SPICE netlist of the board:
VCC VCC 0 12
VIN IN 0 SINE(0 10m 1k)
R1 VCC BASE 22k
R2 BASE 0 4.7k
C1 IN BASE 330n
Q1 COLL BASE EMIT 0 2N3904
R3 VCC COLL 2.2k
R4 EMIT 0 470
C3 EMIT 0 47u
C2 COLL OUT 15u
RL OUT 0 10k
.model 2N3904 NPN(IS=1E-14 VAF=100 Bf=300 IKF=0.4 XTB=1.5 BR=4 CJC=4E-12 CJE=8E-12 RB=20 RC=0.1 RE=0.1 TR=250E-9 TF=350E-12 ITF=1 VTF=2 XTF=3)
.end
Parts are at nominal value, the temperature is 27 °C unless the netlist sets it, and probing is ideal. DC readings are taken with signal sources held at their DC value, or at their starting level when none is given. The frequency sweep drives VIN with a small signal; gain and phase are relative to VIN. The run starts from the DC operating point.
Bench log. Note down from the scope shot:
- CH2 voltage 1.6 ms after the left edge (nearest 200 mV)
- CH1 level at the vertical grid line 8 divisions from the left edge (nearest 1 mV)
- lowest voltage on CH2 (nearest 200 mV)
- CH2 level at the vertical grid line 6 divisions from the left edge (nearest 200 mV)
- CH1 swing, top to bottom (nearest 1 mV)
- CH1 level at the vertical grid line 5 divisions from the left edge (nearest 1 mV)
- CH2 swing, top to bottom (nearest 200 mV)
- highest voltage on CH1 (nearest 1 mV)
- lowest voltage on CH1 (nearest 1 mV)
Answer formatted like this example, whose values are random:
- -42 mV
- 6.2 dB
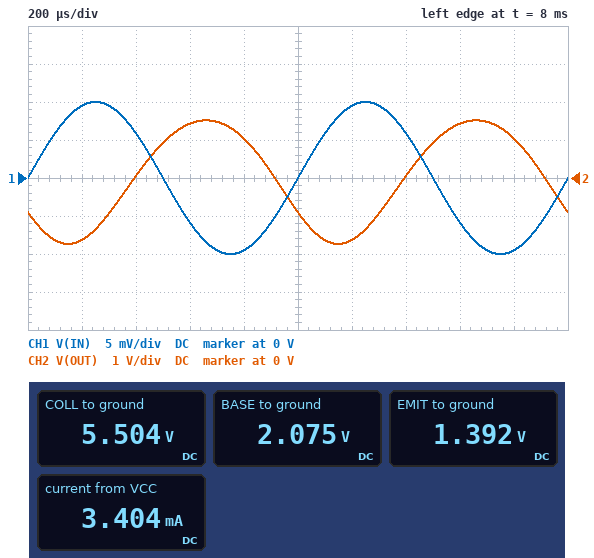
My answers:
- 1.4 V
- -6 mV
- -1.8 V
- -1.6 V
- 20 mV
- 0 V
- 3.2 V
- 10 mV
- -10 mV
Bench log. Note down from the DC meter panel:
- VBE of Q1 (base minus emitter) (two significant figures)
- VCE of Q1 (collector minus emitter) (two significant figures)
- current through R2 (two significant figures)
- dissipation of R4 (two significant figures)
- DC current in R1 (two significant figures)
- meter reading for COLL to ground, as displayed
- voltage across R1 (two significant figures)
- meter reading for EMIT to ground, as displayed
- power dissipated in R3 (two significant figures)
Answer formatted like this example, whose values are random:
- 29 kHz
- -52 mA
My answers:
- 680 mV
- 4.1 V
- 440 µA
- 4.1 mW
- 450 µA
- 5.504 V
- 9.9 V
- 1.392 V
- 19 mW
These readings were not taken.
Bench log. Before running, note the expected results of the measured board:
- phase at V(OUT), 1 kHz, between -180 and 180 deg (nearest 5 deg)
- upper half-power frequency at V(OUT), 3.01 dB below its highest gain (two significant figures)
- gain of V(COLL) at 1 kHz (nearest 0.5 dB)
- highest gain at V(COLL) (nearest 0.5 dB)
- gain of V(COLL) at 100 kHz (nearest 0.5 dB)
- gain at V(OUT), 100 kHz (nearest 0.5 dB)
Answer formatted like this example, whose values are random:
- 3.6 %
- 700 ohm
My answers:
- -145 deg
- 12 MHz
- 44.5 dB
- 45.5 dB
- 45.5 dB
- 45.5 dB
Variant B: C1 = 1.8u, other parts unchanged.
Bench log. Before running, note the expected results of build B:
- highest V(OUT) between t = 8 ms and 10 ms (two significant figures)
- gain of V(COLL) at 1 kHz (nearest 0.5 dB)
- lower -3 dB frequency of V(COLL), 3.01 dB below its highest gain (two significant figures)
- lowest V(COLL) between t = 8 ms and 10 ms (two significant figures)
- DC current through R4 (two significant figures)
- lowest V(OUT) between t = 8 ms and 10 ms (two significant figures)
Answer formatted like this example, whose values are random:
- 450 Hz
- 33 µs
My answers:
- 1.6 V
- 45.0 dB
- 400 Hz
- 3.6 V
- 3.0 mA
- -1.9 V
